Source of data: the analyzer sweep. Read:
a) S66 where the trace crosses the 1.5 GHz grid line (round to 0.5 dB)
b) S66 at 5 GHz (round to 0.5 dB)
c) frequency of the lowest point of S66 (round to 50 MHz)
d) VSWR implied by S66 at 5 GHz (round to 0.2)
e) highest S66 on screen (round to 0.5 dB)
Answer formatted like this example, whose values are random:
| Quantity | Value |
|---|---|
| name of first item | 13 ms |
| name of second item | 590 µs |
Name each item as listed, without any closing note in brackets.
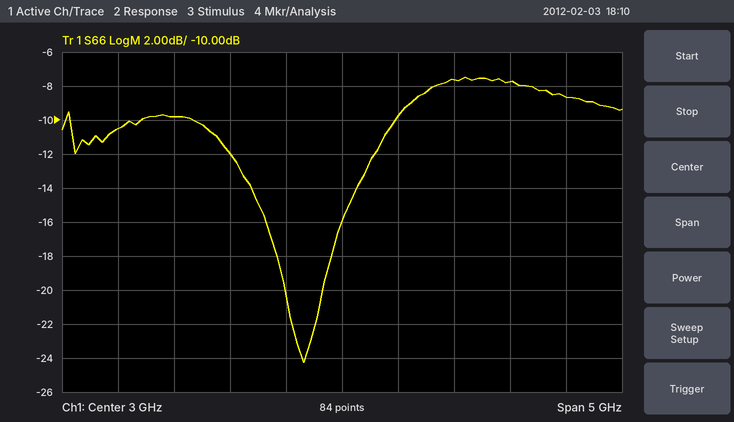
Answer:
| Quantity | Value |
|---|---|
| S66 where the trace crosses the 1.5 GHz grid line | -10.0 dB |
| S66 at 5 GHz | -8.5 dB |
| frequency of the lowest point of S66 | 2.65 GHz |
| VSWR implied by S66 at 5 GHz | 2.2 |
| highest S66 on screen | -7.5 dB |
